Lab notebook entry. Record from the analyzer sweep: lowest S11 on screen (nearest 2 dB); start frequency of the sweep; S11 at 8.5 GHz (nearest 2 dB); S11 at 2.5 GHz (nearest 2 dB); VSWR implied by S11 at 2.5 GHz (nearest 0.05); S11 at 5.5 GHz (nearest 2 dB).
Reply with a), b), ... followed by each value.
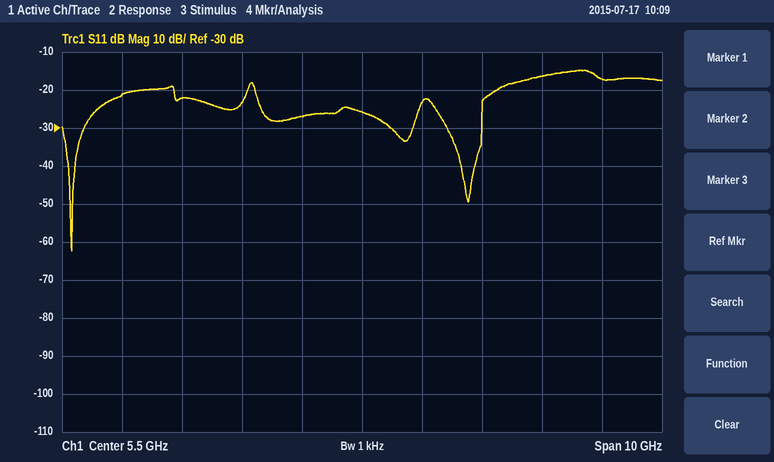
a) -62 dB
b) 500 MHz
c) -16 dB
d) -22 dB
e) 1.15
f) -26 dB
